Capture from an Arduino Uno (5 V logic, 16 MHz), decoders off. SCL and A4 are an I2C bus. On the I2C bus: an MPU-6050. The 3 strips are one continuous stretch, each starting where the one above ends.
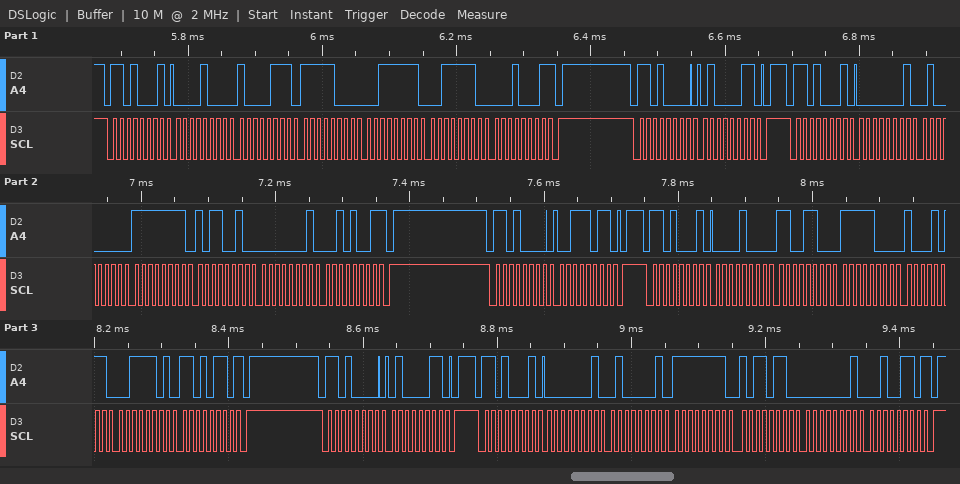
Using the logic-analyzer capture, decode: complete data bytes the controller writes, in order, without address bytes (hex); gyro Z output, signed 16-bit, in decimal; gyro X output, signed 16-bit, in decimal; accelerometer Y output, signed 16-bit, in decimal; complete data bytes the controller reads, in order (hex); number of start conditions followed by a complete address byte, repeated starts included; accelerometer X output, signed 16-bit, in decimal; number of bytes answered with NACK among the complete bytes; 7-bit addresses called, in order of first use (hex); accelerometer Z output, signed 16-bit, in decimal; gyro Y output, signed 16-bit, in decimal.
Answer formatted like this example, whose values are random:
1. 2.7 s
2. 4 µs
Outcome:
1. 43 3B 43
2. 297
3. 320
4. -1909
5. 08 87 F8 3F 3E 11 01 40 FF B2 01 29 08 CC F8 8B 3D D6 01 41 FF B6 01 26
6. 7
7. 2252
8. 4
9. 0x68
10. 15830
11. -78
